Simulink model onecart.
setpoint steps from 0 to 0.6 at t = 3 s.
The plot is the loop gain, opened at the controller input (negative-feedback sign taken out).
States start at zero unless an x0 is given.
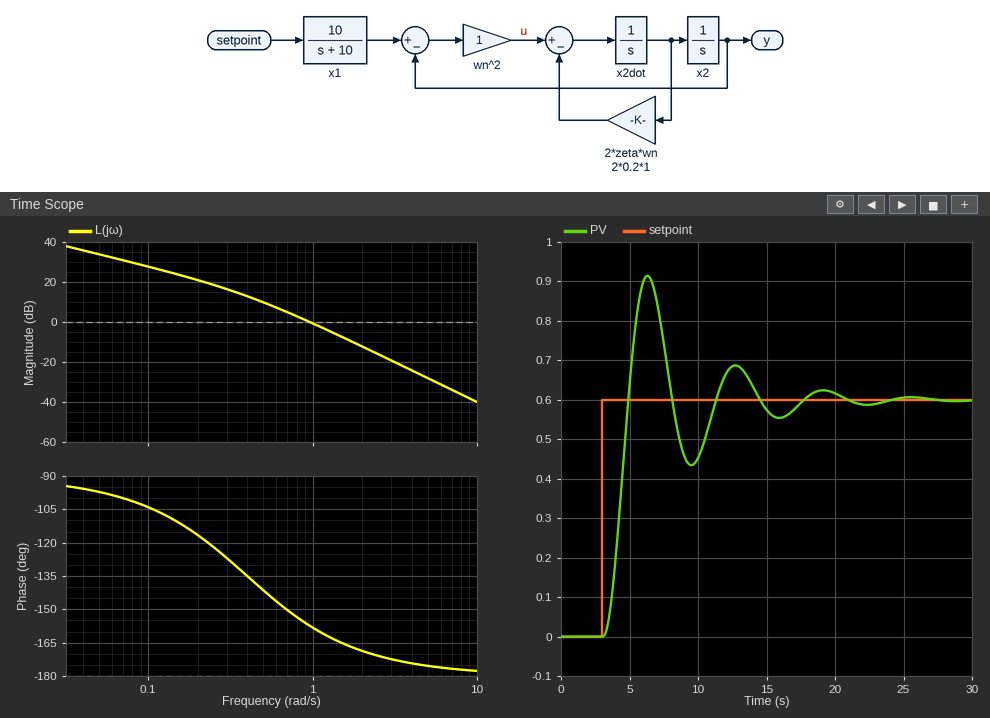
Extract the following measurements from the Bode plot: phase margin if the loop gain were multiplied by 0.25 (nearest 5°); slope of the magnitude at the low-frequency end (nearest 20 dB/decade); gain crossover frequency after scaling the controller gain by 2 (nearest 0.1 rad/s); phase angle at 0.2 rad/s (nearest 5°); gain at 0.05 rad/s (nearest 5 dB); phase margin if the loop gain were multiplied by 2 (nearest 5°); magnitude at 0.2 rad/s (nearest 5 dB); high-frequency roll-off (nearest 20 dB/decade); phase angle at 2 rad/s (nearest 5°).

45°
-20 dB/decade
1.4 rad/s
-115°
35 dB
15°
20 dB
-40 dB/decade
-170°
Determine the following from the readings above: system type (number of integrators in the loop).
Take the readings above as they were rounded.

1
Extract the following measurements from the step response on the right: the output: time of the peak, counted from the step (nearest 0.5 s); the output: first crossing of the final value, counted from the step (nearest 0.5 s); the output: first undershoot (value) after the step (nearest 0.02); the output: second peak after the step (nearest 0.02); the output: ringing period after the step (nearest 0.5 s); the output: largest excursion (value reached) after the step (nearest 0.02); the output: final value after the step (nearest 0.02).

3.5 s
2.0 s
0.44
0.68
6.5 s
0.92
0.60
